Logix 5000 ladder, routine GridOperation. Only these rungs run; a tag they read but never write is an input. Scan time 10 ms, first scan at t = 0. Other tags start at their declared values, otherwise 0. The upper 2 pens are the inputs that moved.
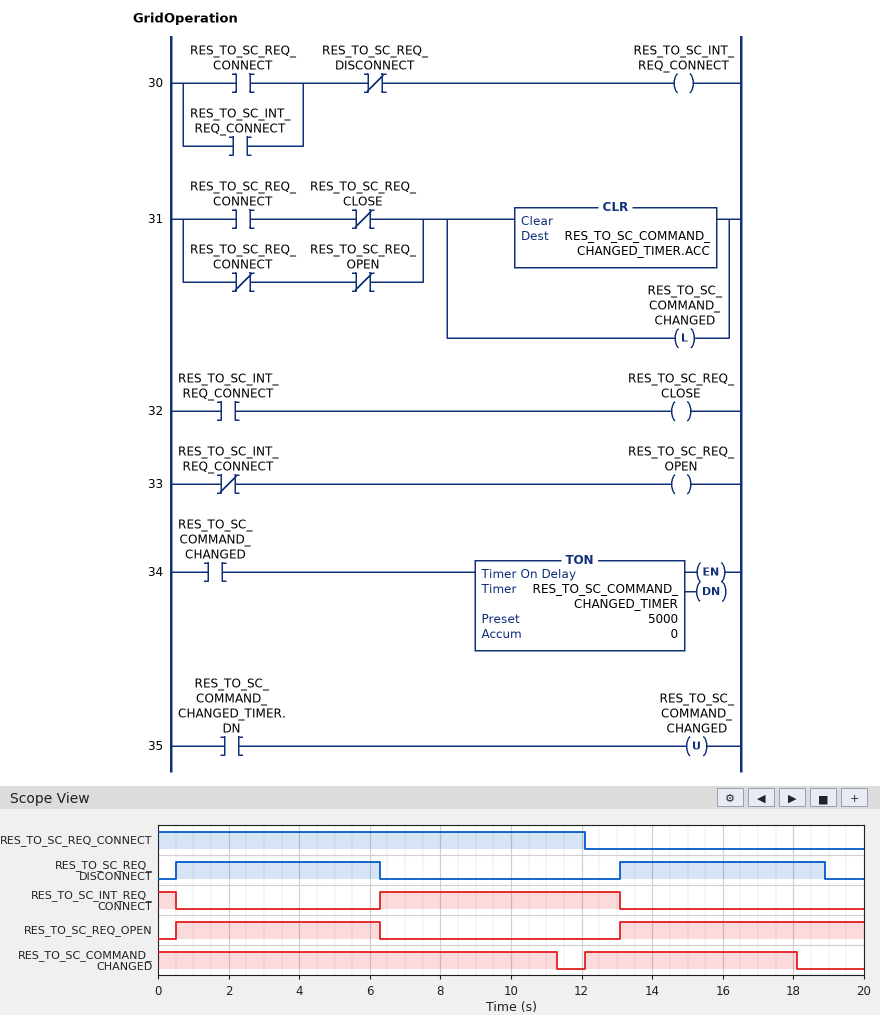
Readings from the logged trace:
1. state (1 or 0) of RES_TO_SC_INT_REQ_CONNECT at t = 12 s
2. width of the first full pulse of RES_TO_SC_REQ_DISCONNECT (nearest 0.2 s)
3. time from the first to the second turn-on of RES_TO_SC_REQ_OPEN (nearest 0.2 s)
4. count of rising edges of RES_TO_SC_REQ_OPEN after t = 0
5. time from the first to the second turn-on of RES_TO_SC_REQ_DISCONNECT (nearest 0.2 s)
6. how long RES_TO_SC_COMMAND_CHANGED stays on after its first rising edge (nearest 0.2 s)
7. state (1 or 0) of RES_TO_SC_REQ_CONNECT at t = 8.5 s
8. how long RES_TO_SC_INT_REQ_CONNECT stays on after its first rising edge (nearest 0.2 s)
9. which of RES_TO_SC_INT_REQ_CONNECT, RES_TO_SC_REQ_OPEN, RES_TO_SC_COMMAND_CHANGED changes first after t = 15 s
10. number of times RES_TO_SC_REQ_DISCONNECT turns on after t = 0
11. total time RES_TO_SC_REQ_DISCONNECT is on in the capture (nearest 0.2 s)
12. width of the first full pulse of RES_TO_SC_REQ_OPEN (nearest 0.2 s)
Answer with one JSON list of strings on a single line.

["1", "5.8 s", "12.6 s", "2", "12.6 s", "6.0 s", "1", "6.8 s", "RES_TO_SC_COMMAND_CHANGED", "2", "11.6 s", "5.8 s"]
